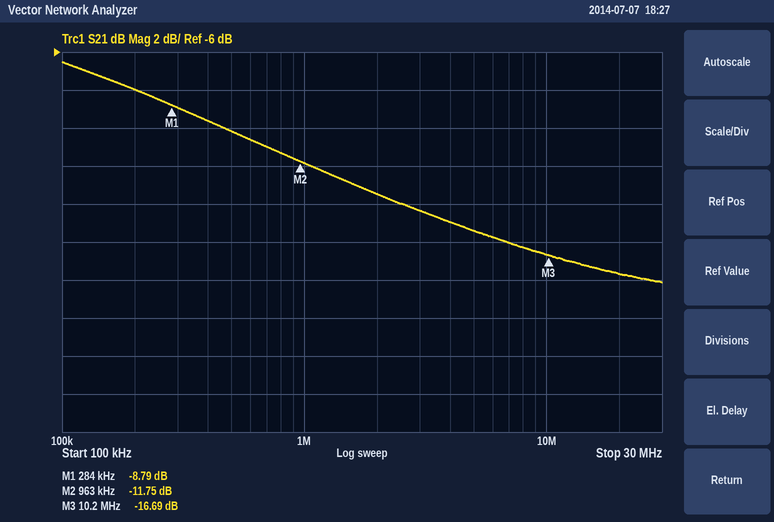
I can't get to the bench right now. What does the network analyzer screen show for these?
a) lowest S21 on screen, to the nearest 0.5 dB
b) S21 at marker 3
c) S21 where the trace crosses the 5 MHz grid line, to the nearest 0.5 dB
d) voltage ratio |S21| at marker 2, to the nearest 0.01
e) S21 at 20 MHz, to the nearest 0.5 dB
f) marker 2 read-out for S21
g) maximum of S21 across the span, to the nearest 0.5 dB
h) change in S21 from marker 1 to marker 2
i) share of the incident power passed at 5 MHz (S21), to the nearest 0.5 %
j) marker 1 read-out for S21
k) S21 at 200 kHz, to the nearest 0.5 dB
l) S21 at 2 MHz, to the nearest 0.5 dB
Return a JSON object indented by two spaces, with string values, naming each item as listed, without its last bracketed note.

{
  "lowest S21 on screen, to the nearest 0.5 dB": "-18.0 dB",
  "S21 at marker 3": "-16.69 dB",
  "S21 where the trace crosses the 5 MHz grid line, to the nearest 0.5 dB": "-15.5 dB",
  "voltage ratio |S21| at marker 2, to the nearest 0.01": "0.26",
  "S21 at 20 MHz, to the nearest 0.5 dB": "-17.5 dB",
  "marker 2 read-out for S21": "-11.75 dB",
  "maximum of S21 across the span, to the nearest 0.5 dB": "-6.5 dB",
  "change in S21 from marker 1 to marker 2": "-2.96 dB",
  "share of the incident power passed at 5 MHz (S21), to the nearest 0.5 %": "3.0 %",
  "marker 1 read-out for S21": "-8.79 dB",
  "S21 at 200 kHz, to the nearest 0.5 dB": "-8.0 dB",
  "S21 at 2 MHz, to the nearest 0.5 dB": "-13.5 dB"
}
